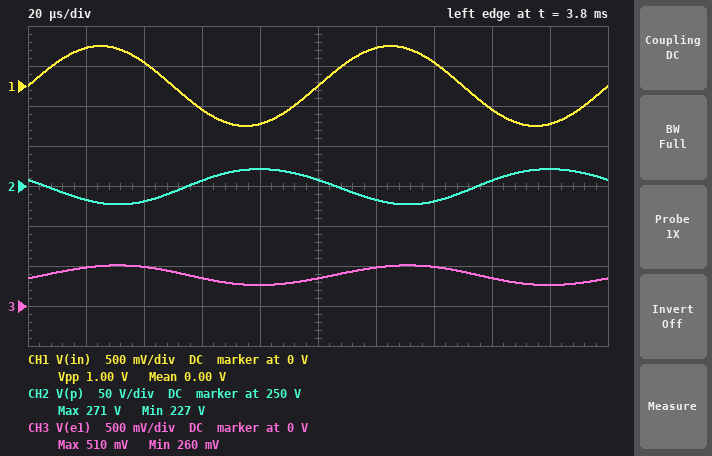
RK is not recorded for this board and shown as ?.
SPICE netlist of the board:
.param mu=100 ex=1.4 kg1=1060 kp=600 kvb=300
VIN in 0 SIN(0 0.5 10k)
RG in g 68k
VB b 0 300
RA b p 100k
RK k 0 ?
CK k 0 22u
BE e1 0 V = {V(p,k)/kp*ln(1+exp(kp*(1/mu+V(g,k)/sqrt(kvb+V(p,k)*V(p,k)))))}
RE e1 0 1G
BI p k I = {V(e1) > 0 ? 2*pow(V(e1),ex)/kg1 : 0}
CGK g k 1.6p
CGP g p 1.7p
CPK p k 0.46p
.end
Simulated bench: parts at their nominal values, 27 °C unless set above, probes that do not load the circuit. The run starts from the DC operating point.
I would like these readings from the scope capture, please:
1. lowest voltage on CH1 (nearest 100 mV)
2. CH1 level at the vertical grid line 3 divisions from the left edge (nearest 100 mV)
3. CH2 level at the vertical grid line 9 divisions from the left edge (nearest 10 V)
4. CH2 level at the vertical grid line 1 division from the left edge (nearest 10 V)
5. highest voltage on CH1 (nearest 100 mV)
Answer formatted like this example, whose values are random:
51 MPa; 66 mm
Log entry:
-500 mV; -300 mV; 270 V; 230 V; 500 mV
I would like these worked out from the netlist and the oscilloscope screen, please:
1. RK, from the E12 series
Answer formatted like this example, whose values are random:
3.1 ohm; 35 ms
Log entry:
4.7 kΩ
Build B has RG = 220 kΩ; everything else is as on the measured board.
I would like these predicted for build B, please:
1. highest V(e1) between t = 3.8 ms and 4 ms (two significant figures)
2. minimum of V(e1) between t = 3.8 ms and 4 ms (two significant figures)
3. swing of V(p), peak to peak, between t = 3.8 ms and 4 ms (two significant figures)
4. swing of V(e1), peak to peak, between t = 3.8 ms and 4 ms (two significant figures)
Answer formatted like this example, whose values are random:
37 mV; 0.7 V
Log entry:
470 mV; 300 mV; 31 V; 170 mV
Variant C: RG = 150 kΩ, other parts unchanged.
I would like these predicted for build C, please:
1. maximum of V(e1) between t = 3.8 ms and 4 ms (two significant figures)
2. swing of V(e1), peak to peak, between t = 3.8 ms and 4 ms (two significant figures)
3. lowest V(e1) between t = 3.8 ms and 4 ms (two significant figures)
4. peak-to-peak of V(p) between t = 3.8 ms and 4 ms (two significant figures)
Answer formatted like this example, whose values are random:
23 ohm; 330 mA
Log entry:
490 mV; 210 mV; 280 mV; 37 V
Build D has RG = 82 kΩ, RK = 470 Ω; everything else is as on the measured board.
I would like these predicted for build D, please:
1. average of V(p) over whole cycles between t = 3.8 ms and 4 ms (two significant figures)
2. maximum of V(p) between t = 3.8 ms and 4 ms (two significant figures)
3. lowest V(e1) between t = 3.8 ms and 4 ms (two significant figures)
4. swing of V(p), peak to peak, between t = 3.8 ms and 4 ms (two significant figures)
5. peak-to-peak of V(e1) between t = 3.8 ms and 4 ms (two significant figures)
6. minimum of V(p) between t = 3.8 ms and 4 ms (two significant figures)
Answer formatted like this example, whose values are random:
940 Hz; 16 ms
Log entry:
150 V; 180 V; 720 mV; 58 V; 240 mV; 120 V
